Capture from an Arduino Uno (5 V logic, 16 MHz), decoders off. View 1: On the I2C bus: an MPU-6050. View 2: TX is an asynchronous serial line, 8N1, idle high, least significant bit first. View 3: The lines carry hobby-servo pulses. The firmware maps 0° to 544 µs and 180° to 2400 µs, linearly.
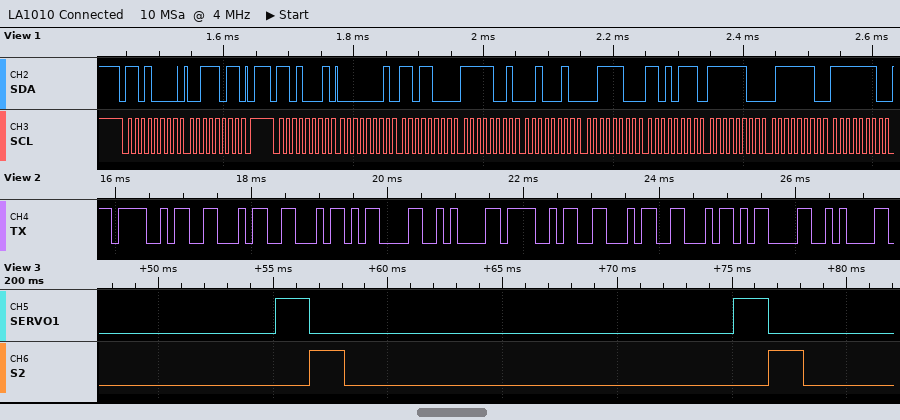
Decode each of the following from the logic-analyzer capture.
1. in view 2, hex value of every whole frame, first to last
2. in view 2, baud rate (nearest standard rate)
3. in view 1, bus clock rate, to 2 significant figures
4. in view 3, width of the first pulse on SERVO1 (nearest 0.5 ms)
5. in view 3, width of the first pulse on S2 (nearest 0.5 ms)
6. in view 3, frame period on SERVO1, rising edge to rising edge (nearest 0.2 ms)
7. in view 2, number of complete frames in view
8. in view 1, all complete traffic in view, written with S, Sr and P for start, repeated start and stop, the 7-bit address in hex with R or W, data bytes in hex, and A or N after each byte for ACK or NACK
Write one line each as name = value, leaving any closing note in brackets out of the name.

in view 2, hex value of every whole frame, first to last = 4F 46 46 0D 0A 4F 46 46 0D 0A
in view 2, baud rate = 9600 baud
in view 1, bus clock rate, to 2 significant figures = 100 kHz
in view 3, width of the first pulse on SERVO1 = 1.5 ms
in view 3, width of the first pulse on S2 = 1.5 ms
in view 3, frame period on SERVO1, rising edge to rising edge = 20.0 ms
in view 2, number of complete frames in view = 10
in view 1, all complete traffic in view, written with S, Sr and P for start, repeated start and stop, the 7-bit address in hex with R or W, data bytes in hex, and A or N after each byte for ACK or NACK = S 68W A 3B A P S 68R A 01 A D8 A F9 A 22 A 3C A D7 A FC A 7E A FE A
